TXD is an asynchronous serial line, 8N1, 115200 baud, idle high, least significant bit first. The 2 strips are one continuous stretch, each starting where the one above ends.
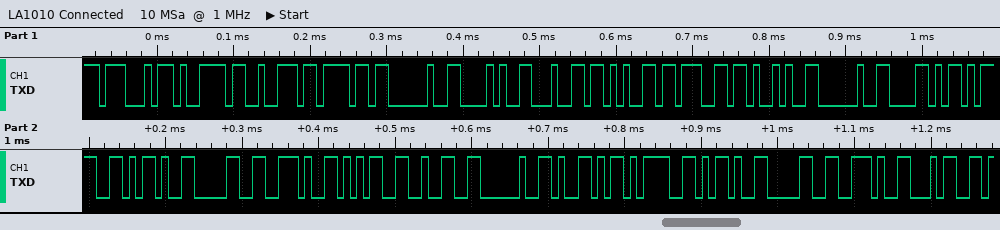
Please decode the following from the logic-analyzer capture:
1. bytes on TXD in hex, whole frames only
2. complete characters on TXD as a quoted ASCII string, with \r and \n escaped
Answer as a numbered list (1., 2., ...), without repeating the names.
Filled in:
1. 47 79 72 6F 20 28 64 65 67 29 20 58 3D 2D 30 2E 35 32 20 59 3D 2D 30 2E 34
2. "Gyro (deg) X=-0.52 Y=-0.4"
